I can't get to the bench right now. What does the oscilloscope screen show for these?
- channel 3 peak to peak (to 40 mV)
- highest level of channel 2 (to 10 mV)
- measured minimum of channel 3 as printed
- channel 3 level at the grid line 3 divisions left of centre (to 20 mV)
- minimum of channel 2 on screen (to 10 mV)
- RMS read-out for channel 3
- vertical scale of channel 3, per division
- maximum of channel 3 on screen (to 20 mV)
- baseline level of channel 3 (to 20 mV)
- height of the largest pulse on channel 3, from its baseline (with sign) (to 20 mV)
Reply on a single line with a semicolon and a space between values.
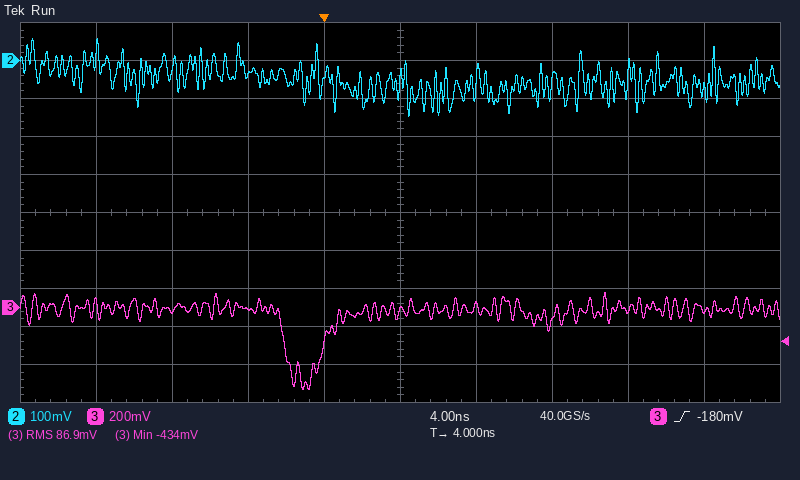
520 mV; 60 mV; -434 mV; -20 mV; -150 mV; 86.9 mV; 200 mV; 80 mV; -20 mV; -420 mV
